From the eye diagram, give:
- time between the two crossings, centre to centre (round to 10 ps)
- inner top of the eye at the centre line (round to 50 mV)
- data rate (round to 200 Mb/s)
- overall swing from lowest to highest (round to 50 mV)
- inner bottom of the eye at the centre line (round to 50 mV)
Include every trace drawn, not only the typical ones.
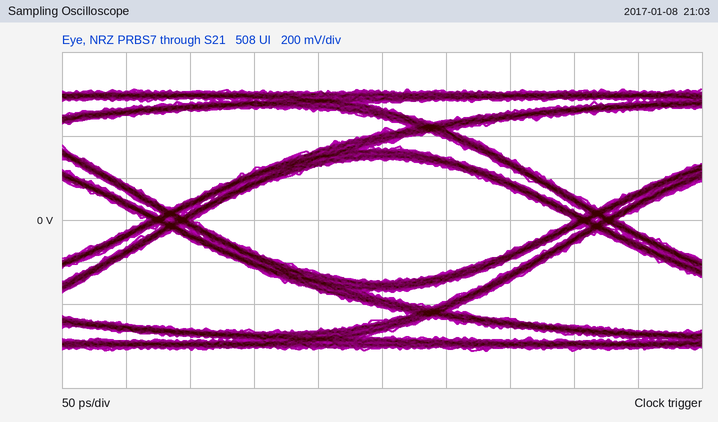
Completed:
330 ps
300 mV
3.0 Gb/s
1.25 V
-300 mV
